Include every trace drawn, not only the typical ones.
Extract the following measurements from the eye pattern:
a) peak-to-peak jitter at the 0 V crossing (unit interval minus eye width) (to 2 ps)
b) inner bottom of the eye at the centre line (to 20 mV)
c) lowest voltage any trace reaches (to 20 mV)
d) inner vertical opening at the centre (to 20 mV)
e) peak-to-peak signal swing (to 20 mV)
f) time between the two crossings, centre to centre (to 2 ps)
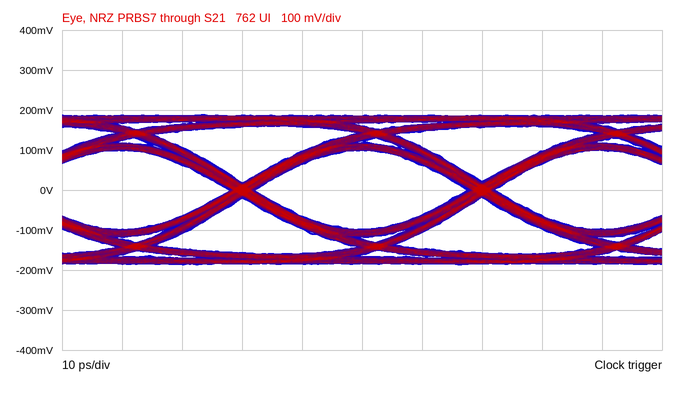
4 ps
-100 mV
-180 mV
200 mV
380 mV
40 ps
